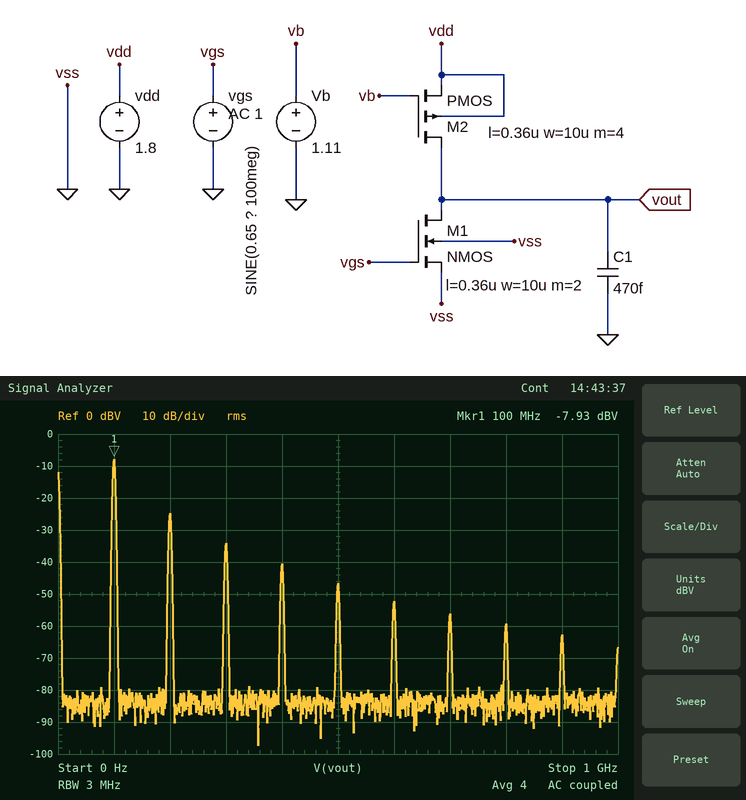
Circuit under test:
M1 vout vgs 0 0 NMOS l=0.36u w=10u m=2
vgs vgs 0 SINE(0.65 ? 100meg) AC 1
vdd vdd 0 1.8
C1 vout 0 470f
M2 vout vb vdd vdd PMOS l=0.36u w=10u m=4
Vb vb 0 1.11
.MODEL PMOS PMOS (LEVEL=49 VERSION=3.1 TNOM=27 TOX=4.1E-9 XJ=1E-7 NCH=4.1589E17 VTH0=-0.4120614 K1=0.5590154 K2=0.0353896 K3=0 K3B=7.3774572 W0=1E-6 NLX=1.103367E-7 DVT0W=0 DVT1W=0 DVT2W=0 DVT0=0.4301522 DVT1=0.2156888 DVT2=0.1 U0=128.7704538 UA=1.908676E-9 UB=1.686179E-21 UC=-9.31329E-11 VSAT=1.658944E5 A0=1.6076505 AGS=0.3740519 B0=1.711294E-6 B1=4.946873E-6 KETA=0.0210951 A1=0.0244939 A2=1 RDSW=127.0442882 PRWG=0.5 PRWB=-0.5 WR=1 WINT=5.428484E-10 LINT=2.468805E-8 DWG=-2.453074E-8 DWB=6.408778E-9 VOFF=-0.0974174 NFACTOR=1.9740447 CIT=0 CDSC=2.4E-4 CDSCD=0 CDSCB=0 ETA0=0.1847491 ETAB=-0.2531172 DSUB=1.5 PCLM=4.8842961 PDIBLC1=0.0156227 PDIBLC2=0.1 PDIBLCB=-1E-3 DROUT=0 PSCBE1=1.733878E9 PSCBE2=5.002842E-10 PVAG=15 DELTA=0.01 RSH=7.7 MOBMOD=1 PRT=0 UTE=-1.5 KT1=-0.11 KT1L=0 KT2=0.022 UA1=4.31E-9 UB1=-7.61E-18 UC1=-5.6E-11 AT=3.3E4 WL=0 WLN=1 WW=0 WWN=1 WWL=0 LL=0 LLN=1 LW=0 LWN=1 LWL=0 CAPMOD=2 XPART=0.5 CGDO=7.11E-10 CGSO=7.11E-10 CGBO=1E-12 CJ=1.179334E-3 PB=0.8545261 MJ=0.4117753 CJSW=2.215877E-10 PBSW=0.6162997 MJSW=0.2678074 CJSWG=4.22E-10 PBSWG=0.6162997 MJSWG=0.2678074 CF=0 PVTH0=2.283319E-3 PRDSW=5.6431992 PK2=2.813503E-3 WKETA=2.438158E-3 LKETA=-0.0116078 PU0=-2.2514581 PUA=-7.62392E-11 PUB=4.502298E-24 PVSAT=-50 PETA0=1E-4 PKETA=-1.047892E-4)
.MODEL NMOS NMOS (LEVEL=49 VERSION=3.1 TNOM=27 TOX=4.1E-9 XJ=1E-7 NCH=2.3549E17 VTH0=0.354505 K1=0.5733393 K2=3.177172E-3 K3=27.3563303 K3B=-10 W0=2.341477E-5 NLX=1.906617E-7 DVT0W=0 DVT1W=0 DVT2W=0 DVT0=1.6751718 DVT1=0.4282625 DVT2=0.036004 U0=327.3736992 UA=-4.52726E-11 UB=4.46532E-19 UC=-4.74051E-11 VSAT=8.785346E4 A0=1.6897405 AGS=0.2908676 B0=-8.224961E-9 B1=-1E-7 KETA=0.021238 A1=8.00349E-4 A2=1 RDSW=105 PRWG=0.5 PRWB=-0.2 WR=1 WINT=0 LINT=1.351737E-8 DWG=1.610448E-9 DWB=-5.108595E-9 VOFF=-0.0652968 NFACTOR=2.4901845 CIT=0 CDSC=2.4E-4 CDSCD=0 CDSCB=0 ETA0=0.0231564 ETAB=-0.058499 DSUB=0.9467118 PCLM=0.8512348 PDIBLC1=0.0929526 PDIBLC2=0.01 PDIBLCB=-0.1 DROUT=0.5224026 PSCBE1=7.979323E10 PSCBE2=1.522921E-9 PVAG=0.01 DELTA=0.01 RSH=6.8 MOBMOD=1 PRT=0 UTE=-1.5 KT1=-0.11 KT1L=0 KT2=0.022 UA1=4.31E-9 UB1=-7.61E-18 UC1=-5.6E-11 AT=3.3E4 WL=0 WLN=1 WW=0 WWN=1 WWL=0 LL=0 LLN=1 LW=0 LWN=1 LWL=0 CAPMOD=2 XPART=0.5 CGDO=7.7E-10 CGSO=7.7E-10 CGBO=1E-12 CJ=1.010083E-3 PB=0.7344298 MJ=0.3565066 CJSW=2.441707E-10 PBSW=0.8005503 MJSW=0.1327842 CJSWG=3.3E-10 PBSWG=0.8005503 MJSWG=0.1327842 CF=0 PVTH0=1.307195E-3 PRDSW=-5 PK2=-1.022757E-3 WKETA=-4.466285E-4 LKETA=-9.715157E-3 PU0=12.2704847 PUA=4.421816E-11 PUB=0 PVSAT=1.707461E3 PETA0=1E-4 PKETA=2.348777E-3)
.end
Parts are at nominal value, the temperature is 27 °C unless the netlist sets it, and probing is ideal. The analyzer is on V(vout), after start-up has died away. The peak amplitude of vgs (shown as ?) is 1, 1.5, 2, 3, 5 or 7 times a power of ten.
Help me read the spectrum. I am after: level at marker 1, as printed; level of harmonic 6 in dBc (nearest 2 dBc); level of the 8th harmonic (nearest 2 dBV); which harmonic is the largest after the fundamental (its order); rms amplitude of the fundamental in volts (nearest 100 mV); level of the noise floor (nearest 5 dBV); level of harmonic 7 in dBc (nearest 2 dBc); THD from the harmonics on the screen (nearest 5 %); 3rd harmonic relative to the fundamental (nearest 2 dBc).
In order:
-7.93 dBV
-44 dBc
-60 dBV
2
400 mV
-85 dBV
-48 dBc
15 %
-26 dBc
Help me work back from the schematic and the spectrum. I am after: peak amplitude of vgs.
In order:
100 mV
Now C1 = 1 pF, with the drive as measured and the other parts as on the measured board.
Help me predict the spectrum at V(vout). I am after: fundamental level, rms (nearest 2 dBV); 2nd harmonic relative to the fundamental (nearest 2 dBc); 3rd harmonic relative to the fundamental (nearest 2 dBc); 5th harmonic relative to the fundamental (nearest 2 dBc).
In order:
-14 dBV
-18 dBc
-32 dBc
-46 dBc
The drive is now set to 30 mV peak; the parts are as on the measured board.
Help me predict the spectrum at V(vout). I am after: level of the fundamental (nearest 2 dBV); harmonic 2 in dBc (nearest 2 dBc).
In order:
-16 dBV
-32 dBc
